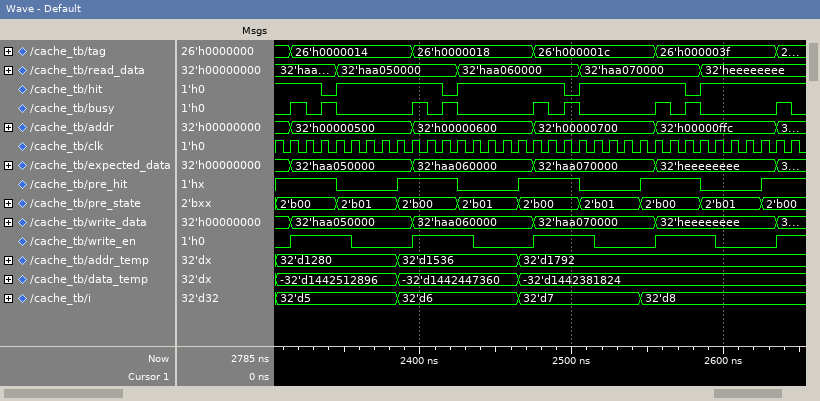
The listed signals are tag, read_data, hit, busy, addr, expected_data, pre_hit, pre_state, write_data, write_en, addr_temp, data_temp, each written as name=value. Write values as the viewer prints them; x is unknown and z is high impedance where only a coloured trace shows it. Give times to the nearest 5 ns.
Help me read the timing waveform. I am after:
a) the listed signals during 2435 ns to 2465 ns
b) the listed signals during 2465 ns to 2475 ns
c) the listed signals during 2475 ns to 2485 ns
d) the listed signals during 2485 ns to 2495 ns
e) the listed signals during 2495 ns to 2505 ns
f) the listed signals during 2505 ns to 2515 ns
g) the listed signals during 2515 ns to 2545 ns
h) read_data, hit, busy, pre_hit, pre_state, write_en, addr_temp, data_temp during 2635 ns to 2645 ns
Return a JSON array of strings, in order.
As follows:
["tag=26'h0000018, read_data=32'haa060000, hit=1, busy=0, addr=32'h00000600, expected_data=32'haa060000, pre_hit=0, pre_state=2'b01, write_data=32'haa060000, write_en=0, addr_temp=32'd1536, data_temp=-32'd1442447360", "tag=26'h0000018, read_data=32'haa060000, hit=1, busy=0, addr=32'h00000600, expected_data=32'haa060000, pre_hit=1, pre_state=2'b00, write_data=32'haa060000, write_en=0, addr_temp=32'd1792, data_temp=-32'd1442381824", "tag=26'h000001c, read_data=32'haa060000, hit=1, busy=1, addr=32'h00000700, expected_data=32'haa070000, pre_hit=1, pre_state=2'b00, write_data=32'haa070000, write_en=1, addr_temp=32'd1792, data_temp=-32'd1442381824", "tag=26'h000001c, read_data=32'haa060000, hit=1, busy=0, addr=32'h00000700, expected_data=32'haa070000, pre_hit=1, pre_state=2'b00, write_data=32'haa070000, write_en=1, addr_temp=32'd1792, data_temp=-32'd1442381824", "tag=26'h000001c, read_data=32'haa060000, hit=0, busy=1, addr=32'h00000700, expected_data=32'haa070000, pre_hit=1, pre_state=2'b00, write_data=32'haa070000, write_en=1, addr_temp=32'd1792, data_temp=-32'd1442381824", "tag=26'h000001c, read_data=32'haa070000, hit=1, busy=0, addr=32'h00000700, expected_data=32'haa070000, pre_hit=0, pre_state=2'b01, write_data=32'haa070000, write_en=1, addr_temp=32'd1792, data_temp=-32'd1442381824", "tag=26'h000001c, read_data=32'haa070000, hit=1, busy=0, addr=32'h00000700, expected_data=32'haa070000, pre_hit=0, pre_state=2'b01, write_data=32'haa070000, write_en=0, addr_temp=32'd1792, data_temp=-32'd1442381824", "read_data=32'heeeeeeee, hit=1, busy=1, pre_hit=1, pre_state=2'b00, write_en=1, addr_temp=32'd1792, data_temp=-32'd1442381824"]
